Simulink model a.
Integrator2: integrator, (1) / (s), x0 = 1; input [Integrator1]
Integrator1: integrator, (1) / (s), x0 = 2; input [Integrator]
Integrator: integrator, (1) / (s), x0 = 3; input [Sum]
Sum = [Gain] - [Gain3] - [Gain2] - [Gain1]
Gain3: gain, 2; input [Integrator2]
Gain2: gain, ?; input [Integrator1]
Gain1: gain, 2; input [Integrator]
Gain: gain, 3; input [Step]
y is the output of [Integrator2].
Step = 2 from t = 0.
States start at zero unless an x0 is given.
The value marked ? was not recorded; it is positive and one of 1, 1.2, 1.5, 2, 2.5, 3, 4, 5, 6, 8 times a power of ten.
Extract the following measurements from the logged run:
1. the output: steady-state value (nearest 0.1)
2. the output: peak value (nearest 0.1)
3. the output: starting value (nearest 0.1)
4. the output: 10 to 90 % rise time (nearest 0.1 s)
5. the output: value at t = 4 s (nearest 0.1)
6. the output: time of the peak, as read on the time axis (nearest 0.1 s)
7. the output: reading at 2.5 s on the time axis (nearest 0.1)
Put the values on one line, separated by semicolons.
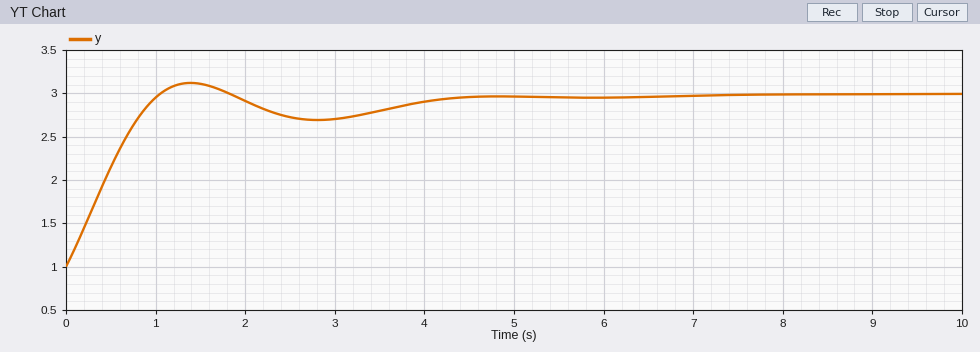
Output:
3.0; 3.1; 1.0; 0.8 s; 2.9; 1.4 s; 2.7
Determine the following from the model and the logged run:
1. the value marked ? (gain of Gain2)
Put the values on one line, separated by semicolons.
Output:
5
